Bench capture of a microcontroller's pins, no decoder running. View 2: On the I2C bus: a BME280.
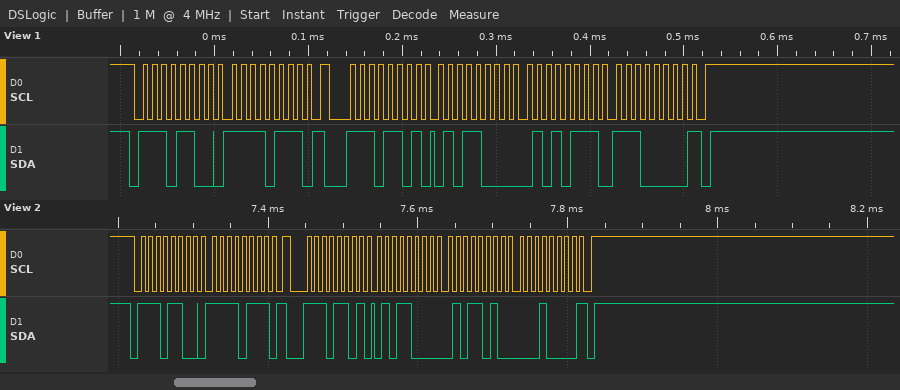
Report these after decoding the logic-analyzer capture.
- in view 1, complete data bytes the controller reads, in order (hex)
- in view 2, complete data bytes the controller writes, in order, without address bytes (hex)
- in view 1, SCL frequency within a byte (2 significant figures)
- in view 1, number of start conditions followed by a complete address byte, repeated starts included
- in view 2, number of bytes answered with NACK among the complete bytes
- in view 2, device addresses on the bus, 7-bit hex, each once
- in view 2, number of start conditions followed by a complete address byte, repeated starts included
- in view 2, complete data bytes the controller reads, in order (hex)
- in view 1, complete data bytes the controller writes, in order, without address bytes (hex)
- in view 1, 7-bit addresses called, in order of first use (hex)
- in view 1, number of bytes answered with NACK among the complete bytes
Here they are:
58 57 E0
F7
100 kHz
2
1
0x76
2
58 5A 10
F7
0x76
1
